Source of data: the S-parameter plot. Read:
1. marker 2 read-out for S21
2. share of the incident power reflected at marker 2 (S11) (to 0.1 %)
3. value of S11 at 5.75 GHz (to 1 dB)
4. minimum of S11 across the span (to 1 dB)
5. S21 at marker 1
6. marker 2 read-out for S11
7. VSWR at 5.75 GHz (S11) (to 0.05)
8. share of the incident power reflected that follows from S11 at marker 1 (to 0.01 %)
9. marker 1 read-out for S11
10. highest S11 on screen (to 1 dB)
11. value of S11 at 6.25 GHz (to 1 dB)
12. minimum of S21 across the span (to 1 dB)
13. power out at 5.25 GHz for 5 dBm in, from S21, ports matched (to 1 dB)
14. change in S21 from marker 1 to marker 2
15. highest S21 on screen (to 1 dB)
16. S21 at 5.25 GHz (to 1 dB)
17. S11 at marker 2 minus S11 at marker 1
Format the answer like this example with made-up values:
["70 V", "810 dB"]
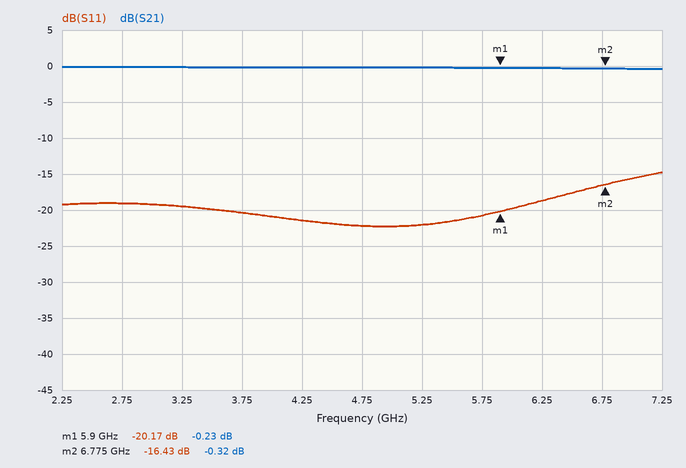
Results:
["-0.32 dB", "2.3 %", "-21 dB", "-22 dB", "-0.23 dB", "-16.43 dB", "1.20", "0.96 %", "-20.17 dB", "-15 dB", "-19 dB", "0 dB", "5 dBm", "-0.09 dB", "0 dB", "0 dB", "3.74 dB"]
